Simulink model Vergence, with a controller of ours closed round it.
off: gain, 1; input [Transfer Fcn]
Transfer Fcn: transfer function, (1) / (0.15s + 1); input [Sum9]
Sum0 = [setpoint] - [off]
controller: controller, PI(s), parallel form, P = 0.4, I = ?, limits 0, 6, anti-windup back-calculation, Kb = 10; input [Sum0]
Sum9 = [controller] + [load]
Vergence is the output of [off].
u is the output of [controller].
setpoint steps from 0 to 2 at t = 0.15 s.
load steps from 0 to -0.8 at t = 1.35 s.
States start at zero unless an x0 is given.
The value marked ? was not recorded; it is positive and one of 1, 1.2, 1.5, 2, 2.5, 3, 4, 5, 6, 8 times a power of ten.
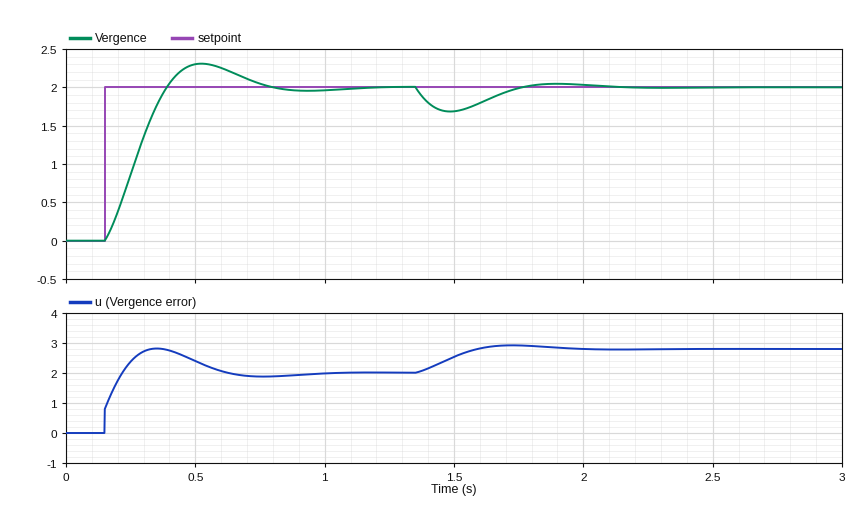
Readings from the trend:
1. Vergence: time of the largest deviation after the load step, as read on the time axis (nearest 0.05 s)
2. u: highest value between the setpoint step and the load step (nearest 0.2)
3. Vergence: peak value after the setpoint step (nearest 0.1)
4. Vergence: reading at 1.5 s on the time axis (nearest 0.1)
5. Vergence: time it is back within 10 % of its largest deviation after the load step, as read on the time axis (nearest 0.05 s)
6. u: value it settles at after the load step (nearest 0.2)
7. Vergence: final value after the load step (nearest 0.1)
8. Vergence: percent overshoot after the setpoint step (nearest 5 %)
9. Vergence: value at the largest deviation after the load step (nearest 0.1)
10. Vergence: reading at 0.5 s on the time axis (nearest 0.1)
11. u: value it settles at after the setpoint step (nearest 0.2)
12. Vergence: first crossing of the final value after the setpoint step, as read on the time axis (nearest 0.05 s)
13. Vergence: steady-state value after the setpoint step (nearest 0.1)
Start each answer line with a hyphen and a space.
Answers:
- 1.50 s
- 2.8
- 2.3
- 1.7
- 2.00 s
- 2.8
- 2.0
- 15 %
- 1.7
- 2.3
- 2.0
- 0.40 s
- 2.0
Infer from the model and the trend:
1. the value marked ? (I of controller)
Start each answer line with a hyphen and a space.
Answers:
- 12
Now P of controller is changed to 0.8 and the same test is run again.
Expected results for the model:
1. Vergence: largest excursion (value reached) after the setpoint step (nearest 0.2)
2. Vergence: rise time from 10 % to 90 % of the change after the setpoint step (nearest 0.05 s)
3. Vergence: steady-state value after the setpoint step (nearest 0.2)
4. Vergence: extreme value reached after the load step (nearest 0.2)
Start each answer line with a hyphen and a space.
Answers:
- 2.2
- 0.20 s
- 2.0
- 1.8
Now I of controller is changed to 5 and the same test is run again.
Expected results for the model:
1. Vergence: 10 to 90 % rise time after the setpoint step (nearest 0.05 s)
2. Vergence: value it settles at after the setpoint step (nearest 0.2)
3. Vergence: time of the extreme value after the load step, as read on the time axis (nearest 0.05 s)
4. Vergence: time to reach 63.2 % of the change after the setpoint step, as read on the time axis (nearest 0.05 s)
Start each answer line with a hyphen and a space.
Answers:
- 0.40 s
- 2.0
- 1.55 s
- 0.40 s
